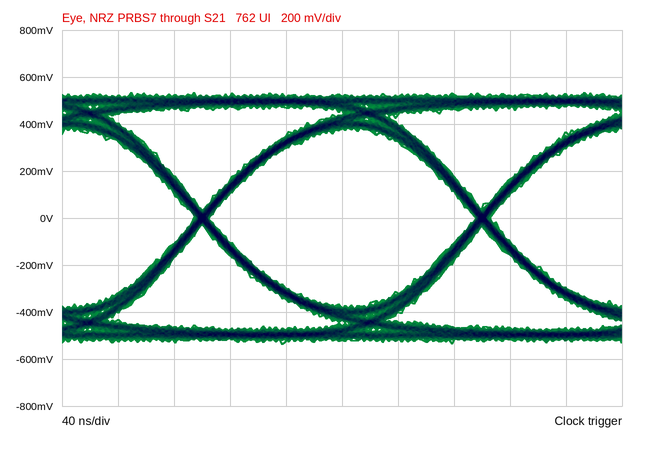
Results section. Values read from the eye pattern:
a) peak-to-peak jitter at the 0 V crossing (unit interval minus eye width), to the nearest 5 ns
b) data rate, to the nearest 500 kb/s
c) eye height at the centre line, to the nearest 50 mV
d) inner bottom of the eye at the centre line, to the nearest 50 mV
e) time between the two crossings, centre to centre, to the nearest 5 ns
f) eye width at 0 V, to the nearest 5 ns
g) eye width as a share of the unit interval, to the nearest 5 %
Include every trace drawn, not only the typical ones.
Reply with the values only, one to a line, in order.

10 ns
5.0 Mb/s
750 mV
-400 mV
200 ns
190 ns
95 %
